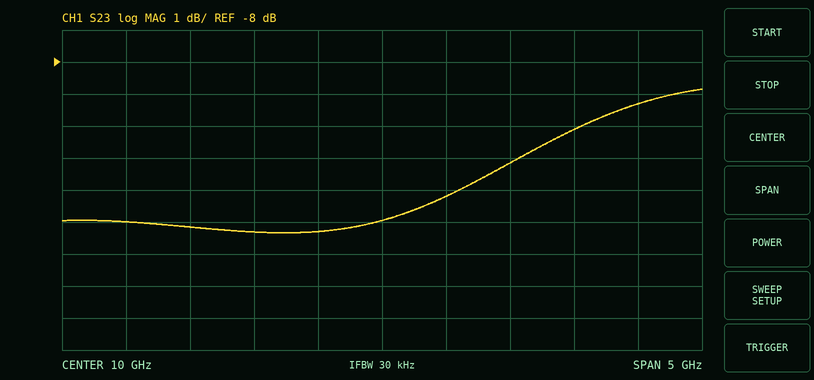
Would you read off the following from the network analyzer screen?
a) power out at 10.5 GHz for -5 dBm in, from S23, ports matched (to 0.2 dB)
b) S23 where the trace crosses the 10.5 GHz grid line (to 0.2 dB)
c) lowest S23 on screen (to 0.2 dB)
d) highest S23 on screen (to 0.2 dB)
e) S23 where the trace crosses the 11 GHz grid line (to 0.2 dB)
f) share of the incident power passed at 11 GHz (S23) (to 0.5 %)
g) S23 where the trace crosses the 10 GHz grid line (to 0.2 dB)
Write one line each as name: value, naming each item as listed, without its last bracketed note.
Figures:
power out at 10.5 GHz for -5 dBm in, from S23, ports matched: -17.2 dBm
S23 where the trace crosses the 10.5 GHz grid line: -12.2 dB
lowest S23 on screen: -13.4 dB
highest S23 on screen: -8.8 dB
S23 where the trace crosses the 11 GHz grid line: -11.2 dB
share of the incident power passed at 11 GHz (S23): 7.5 %
S23 where the trace crosses the 10 GHz grid line: -13.0 dB
